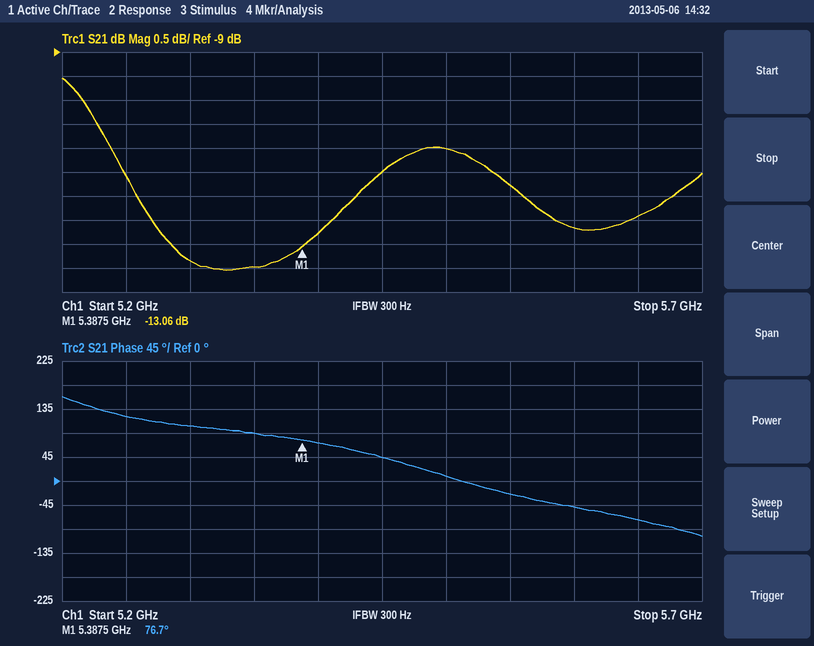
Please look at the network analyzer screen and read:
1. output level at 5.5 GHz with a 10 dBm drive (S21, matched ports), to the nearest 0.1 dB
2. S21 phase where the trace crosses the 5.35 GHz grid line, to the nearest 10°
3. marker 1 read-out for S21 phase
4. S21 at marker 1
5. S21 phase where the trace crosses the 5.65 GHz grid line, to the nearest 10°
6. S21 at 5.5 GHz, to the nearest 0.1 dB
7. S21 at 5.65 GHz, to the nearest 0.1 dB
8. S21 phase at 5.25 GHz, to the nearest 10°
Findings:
-1.0 dBm
90°
76.7°
-13.06 dB
-70°
-11.0 dB
-12.4 dB
120°
